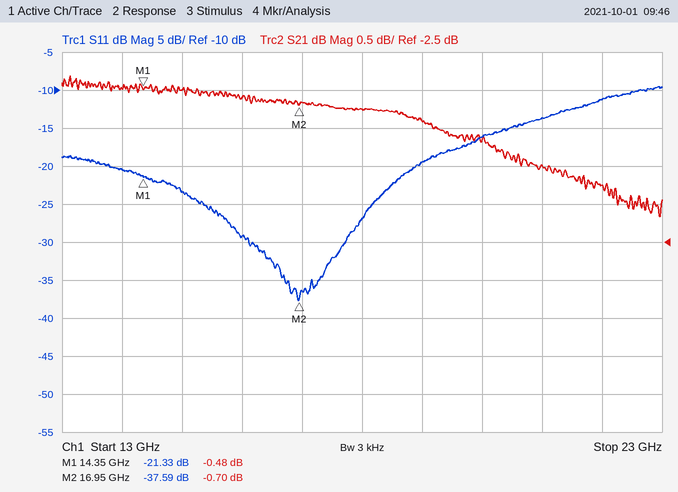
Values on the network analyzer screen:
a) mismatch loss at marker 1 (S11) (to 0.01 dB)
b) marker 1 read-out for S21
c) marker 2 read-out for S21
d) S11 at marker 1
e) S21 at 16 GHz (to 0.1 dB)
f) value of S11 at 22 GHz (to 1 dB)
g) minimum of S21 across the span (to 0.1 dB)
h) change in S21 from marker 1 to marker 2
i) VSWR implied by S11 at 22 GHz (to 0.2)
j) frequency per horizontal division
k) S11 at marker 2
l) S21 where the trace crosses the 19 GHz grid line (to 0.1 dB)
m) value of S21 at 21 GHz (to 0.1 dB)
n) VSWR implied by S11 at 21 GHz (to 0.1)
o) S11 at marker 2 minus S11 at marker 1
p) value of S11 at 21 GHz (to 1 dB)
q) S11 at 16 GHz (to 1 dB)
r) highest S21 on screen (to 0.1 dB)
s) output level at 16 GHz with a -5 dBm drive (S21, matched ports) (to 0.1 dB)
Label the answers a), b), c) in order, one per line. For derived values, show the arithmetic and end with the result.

a) −10 log10(1 − 10^(-21.33/10)) ≈ 0.03 dB
b) -0.48 dB
c) -0.70 dB
d) -21.33 dB
e) -0.6 dB
f) -11 dB
g) -2.2 dB
h) -0.7 − (-0.48) = -0.22 dB
i) |Γ| = 10^(-11/20) = 0.2818; VSWR = (1 + 0.2818)/(1 − 0.2818) ≈ 1.8
j) 1 GHz
k) -37.59 dB
l) -0.9 dB
m) -1.5 dB
n) |Γ| = 10^(-14/20) = 0.1995; VSWR = (1 + 0.1995)/(1 − 0.1995) ≈ 1.5
o) -37.59 − (-21.33) = -16.26 dB
p) -14 dB
q) -29 dB
r) -0.3 dB
s) -5 dBm + (-0.6 dB) = -5.6 dBm
